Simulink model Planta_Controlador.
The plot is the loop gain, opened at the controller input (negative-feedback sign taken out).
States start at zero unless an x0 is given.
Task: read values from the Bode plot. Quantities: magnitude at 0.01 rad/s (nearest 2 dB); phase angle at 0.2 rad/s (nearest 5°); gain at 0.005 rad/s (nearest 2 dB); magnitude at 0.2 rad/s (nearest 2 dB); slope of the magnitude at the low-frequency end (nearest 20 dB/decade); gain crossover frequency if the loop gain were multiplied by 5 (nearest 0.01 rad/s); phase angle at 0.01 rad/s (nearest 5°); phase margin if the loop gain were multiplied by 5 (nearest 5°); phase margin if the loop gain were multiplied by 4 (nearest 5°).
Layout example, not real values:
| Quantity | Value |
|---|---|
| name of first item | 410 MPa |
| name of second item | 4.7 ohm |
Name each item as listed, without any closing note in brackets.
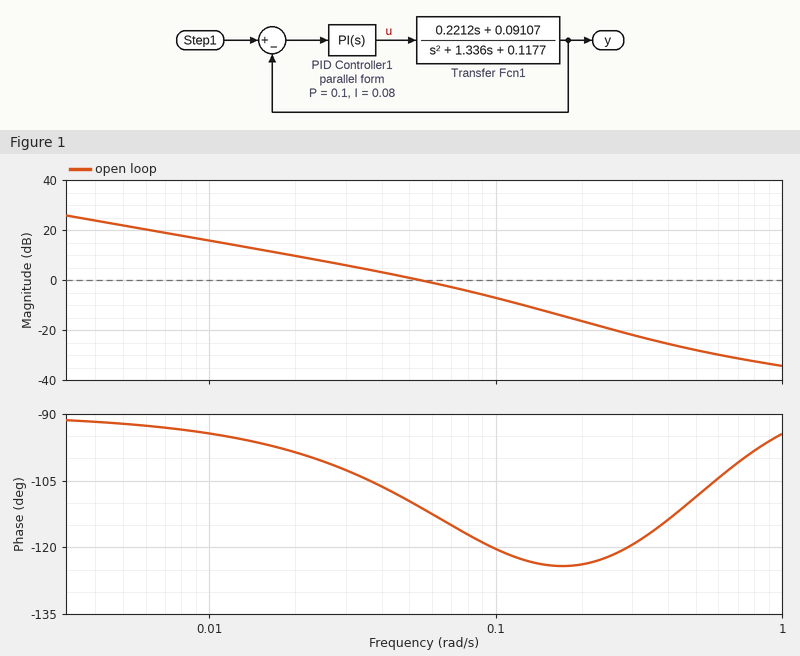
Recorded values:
| Quantity | Value |
|---|---|
| magnitude at 0.01 rad/s | 16 dB |
| phase angle at 0.2 rad/s | -125° |
| gain at 0.005 rad/s | 22 dB |
| magnitude at 0.2 rad/s | -16 dB |
| slope of the magnitude at the low-frequency end | -20 dB/decade |
| gain crossover frequency if the loop gain were multiplied by 5 | 0.17 rad/s |
| phase angle at 0.01 rad/s | -95° |
| phase margin if the loop gain were multiplied by 5 | 55° |
| phase margin if the loop gain were multiplied by 4 | 55° |
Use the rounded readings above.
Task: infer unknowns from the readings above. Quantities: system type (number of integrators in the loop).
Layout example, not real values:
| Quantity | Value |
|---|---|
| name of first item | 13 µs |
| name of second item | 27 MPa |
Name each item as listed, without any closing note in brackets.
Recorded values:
| Quantity | Value |
|---|---|
| system type | 1 |
